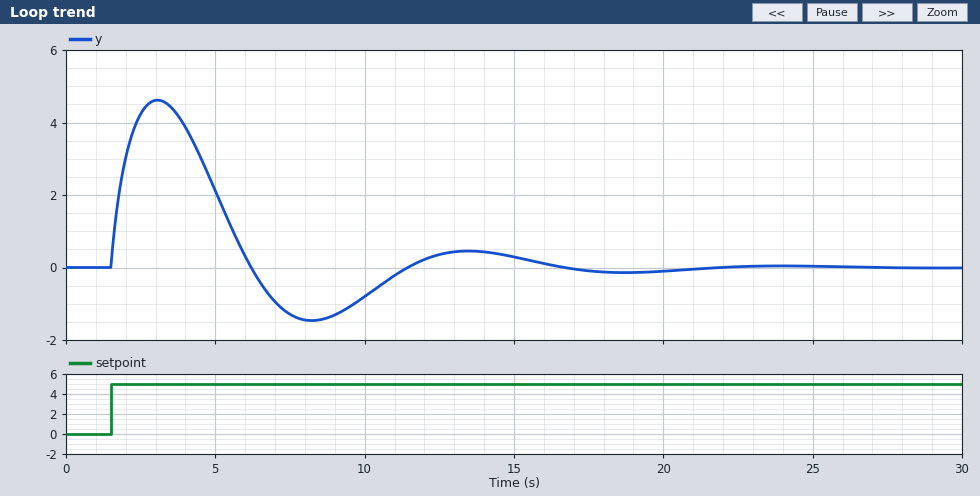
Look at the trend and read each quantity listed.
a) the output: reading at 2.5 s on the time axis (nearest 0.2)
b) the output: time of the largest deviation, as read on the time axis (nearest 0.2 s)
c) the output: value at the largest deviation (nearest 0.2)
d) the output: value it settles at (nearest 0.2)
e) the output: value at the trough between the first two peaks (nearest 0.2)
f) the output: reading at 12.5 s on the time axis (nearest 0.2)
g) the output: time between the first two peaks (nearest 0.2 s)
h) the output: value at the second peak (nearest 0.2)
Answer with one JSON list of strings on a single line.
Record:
["4.2", "3.0 s", "4.6", "0.0", "-1.4", "0.4", "10.4 s", "0.4"]
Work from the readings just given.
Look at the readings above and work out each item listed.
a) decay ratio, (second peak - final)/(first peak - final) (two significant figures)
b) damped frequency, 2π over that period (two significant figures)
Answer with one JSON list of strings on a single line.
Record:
["0.087", "0.60 rad/s"]
